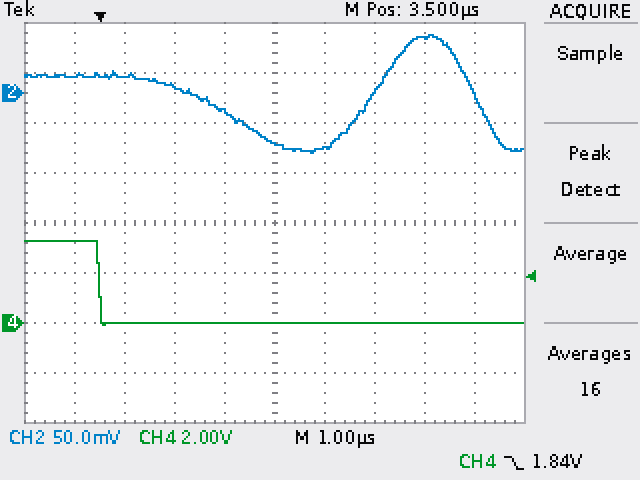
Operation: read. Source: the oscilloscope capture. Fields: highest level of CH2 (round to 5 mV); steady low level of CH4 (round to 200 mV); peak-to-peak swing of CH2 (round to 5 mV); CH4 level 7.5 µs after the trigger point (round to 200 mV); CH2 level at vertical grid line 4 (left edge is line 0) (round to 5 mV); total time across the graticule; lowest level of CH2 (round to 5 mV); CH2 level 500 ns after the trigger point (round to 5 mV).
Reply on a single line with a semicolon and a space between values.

60 mV; 0.0 V; 120 mV; 0.0 V; -20 mV; 10 µs; -60 mV; 15 mV
